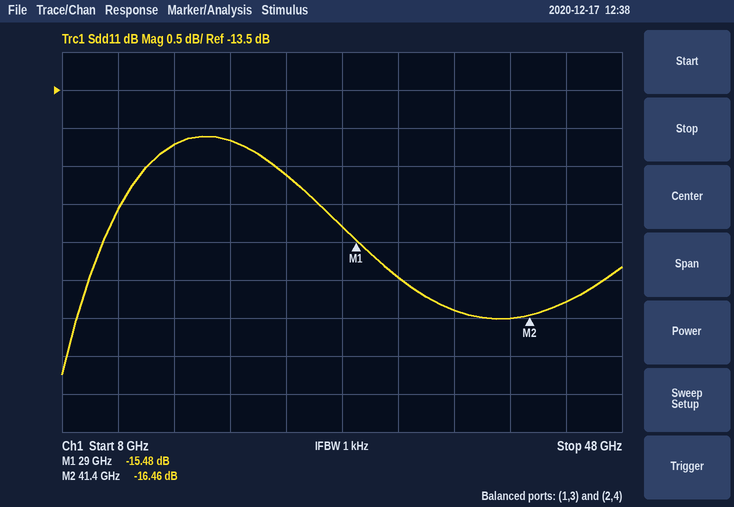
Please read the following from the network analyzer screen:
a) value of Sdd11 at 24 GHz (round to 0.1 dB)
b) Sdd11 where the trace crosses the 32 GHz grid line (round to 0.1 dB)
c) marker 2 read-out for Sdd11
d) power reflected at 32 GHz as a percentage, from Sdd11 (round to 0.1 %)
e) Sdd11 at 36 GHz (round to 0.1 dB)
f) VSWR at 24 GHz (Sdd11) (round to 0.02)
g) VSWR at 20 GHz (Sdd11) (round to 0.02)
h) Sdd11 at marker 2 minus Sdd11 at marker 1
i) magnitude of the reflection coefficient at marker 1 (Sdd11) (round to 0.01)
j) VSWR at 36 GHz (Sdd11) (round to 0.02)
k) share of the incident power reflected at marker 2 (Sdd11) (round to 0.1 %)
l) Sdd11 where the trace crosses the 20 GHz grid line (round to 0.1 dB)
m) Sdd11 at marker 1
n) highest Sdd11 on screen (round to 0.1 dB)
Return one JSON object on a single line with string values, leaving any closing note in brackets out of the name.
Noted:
{"value of Sdd11 at 24 GHz": "-14.6 dB", "Sdd11 where the trace crosses the 32 GHz grid line": "-16.0 dB", "marker 2 read-out for Sdd11": "-16.46 dB", "power reflected at 32 GHz as a percentage, from Sdd11": "2.5 %", "Sdd11 at 36 GHz": "-16.4 dB", "VSWR at 24 GHz (Sdd11)": "1.46", "VSWR at 20 GHz (Sdd11)": "1.48", "Sdd11 at marker 2 minus Sdd11 at marker 1": "-0.98 dB", "magnitude of the reflection coefficient at marker 1 (Sdd11)": "0.17", "VSWR at 36 GHz (Sdd11)": "1.36", "share of the incident power reflected at marker 2 (Sdd11)": "2.3 %", "Sdd11 where the trace crosses the 20 GHz grid line": "-14.2 dB", "Sdd11 at marker 1": "-15.48 dB", "highest Sdd11 on screen": "-14.1 dB"}
